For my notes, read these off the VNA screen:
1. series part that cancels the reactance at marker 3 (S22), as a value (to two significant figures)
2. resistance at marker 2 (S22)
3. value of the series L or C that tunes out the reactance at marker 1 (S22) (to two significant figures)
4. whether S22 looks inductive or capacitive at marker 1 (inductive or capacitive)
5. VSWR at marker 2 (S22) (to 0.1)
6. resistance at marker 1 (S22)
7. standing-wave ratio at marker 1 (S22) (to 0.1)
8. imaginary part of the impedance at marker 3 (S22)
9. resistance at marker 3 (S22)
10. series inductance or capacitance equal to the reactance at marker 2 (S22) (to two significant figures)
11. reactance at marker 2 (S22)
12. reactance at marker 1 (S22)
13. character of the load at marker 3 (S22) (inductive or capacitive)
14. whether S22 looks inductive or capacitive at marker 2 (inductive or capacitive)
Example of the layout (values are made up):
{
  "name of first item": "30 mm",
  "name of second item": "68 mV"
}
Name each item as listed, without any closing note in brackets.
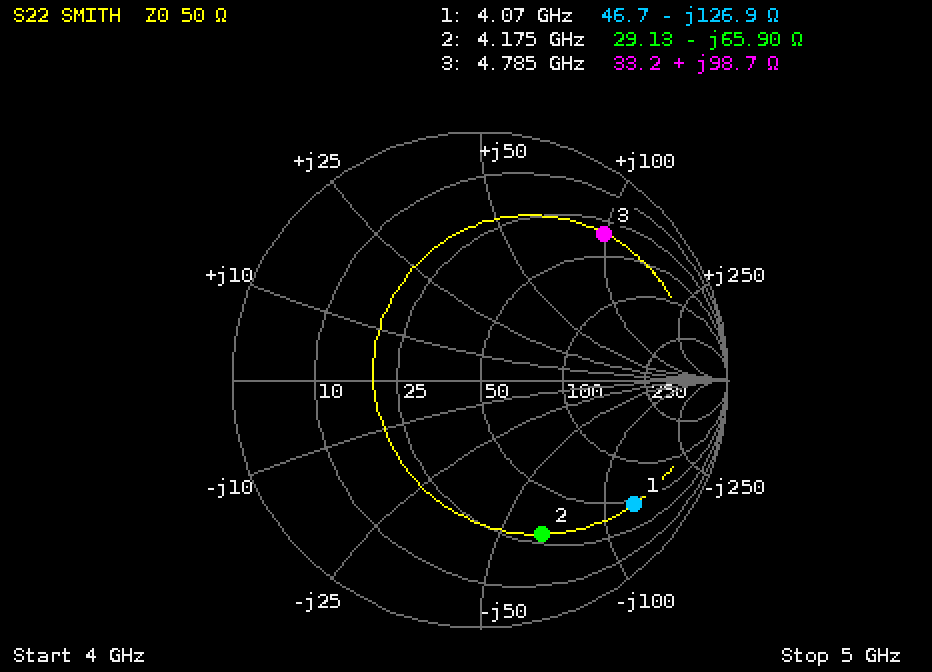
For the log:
{
  "series part that cancels the reactance at marker 3 (S22), as a value": "340 fF",
  "resistance at marker 2": "29.13 Ω",
  "value of the series L or C that tunes out the reactance at marker 1 (S22)": "5.0 nH",
  "whether S22 looks inductive or capacitive at marker 1": "capacitive",
  "VSWR at marker 2 (S22)": "5.1",
  "resistance at marker 1": "46.7 Ω",
  "standing-wave ratio at marker 1 (S22)": "8.8",
  "imaginary part of the impedance at marker 3": "+98.7 Ω",
  "resistance at marker 3": "33.2 Ω",
  "series inductance or capacitance equal to the reactance at marker 2 (S22)": "580 fF",
  "reactance at marker 2": "-65.90 Ω",
  "reactance at marker 1": "-126.9 Ω",
  "character of the load at marker 3 (S22)": "inductive",
  "whether S22 looks inductive or capacitive at marker 2": "capacitive"
}
